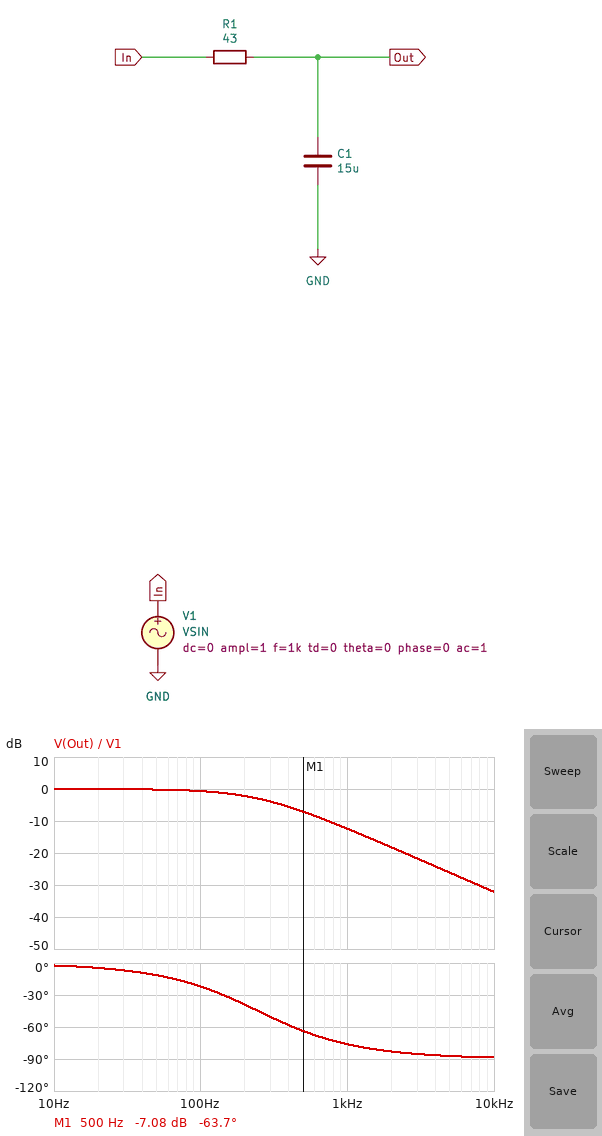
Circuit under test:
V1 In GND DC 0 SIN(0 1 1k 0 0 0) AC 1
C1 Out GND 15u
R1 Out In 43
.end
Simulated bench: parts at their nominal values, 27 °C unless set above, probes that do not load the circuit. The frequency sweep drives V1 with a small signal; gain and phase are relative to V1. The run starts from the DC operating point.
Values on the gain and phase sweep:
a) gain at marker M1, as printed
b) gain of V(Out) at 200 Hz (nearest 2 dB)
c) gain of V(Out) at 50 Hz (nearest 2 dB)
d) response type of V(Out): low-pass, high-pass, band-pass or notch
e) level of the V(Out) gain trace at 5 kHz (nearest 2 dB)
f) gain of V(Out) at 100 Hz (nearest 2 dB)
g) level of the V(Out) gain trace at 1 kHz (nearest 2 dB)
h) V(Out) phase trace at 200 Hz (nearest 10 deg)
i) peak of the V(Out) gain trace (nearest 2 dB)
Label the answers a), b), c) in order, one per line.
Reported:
a) -7.08 dB
b) -2 dB
c) 0 dB
d) low-pass
e) -26 dB
f) 0 dB
g) -12 dB
h) -40 deg
i) 0 dB
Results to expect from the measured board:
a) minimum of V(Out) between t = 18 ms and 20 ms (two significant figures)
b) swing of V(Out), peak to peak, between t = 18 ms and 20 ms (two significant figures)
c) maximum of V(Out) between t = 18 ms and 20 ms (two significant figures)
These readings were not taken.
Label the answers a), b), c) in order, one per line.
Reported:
a) -240 mV
b) 480 mV
c) 240 mV
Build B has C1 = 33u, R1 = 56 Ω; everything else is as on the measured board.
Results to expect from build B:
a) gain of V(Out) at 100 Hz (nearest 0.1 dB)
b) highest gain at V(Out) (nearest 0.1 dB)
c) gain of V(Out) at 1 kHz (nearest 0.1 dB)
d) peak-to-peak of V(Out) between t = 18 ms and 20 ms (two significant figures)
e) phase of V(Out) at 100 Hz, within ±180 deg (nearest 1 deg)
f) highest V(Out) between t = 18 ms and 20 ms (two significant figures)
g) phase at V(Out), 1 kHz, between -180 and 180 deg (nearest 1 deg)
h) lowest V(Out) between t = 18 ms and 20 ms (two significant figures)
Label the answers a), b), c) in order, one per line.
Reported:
a) -3.7 dB
b) 0 dB
c) -21.3 dB
d) 170 mV
e) -49 deg
f) 86 mV
g) -85 deg
h) -86 mV
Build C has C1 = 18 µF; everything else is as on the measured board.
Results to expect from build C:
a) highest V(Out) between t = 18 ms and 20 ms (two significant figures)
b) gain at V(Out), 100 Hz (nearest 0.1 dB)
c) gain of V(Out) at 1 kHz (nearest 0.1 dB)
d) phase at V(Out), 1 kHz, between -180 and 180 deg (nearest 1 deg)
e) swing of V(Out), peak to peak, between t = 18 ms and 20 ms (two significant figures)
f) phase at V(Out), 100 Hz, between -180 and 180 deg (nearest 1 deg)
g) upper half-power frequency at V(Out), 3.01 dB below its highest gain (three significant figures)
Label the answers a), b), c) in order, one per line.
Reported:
a) 200 mV
b) -0.9 dB
c) -13.9 dB
d) -78 deg
e) 400 mV
f) -26 deg
g) 206 Hz
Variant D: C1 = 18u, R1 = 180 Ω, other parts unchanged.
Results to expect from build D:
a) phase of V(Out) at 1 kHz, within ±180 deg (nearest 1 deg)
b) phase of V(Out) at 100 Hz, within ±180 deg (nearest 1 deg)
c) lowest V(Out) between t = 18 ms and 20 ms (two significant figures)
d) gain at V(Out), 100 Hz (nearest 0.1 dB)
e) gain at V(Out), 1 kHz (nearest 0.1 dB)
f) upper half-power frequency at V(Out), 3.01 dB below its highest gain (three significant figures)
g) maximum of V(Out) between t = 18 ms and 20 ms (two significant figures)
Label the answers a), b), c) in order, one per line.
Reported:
a) -87 deg
b) -64 deg
c) -49 mV
d) -7.1 dB
e) -26.2 dB
f) 49.1 Hz
g) 49 mV
